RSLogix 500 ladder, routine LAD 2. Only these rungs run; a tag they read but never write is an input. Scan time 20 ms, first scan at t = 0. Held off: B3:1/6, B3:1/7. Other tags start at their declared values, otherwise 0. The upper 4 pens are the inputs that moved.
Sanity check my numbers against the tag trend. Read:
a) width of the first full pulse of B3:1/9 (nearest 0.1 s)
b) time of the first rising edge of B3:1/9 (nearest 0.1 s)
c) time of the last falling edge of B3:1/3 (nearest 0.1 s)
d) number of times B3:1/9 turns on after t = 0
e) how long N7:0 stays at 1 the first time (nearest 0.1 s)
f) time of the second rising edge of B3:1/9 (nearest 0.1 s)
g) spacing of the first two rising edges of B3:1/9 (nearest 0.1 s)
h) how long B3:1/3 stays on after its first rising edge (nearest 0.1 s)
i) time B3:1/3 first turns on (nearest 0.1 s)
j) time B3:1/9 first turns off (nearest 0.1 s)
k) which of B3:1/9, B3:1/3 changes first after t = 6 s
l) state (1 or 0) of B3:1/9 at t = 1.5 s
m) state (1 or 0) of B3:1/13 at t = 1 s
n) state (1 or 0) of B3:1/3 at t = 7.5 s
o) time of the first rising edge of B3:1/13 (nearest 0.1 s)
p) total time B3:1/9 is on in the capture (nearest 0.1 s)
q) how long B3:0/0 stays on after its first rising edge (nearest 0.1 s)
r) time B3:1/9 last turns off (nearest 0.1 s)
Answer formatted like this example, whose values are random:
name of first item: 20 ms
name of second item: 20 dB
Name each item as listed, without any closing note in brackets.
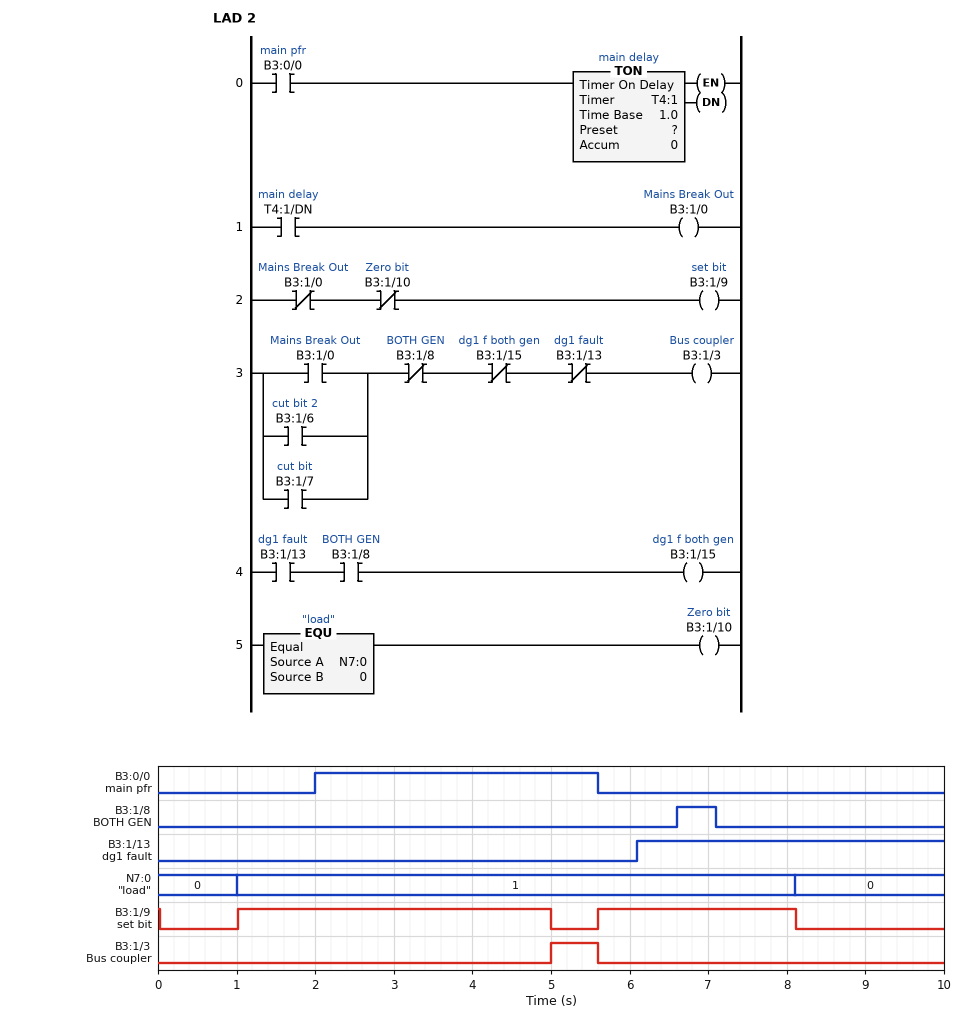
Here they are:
width of the first full pulse of B3:1/9: 4.0 s
time of the first rising edge of B3:1/9: 1.0 s
time of the last falling edge of B3:1/3: 5.6 s
number of times B3:1/9 turns on after t = 0: 2
how long N7:0 stays at 1 the first time: 7.1 s
time of the second rising edge of B3:1/9: 5.6 s
spacing of the first two rising edges of B3:1/9: 4.6 s
how long B3:1/3 stays on after its first rising edge: 0.6 s
time B3:1/3 first turns on: 5.0 s
time B3:1/9 first turns off: 0.0 s
which of B3:1/9, B3:1/3 changes first after t = 6 s: B3:1/9
state (1 or 0) of B3:1/9 at t = 1.5 s: 1
state (1 or 0) of B3:1/13 at t = 1 s: 0
state (1 or 0) of B3:1/3 at t = 7.5 s: 0
time of the first rising edge of B3:1/13: 6.1 s
total time B3:1/9 is on in the capture: 6.5 s
how long B3:0/0 stays on after its first rising edge: 3.6 s
time B3:1/9 last turns off: 8.1 s
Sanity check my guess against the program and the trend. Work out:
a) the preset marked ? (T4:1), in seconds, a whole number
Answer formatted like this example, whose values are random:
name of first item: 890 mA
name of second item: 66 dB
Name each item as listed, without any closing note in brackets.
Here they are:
the preset marked ? (T4:1), in seconds, a whole number: 3 s
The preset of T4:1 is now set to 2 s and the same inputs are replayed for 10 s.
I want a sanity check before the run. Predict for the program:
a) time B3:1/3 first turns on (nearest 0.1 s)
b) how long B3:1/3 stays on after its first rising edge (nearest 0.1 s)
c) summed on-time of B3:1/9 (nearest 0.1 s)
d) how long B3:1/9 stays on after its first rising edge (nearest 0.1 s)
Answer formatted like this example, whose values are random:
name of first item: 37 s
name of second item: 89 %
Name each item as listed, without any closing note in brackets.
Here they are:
time B3:1/3 first turns on: 4.0 s
how long B3:1/3 stays on after its first rising edge: 1.6 s
summed on-time of B3:1/9: 5.5 s
how long B3:1/9 stays on after its first rising edge: 3.0 s
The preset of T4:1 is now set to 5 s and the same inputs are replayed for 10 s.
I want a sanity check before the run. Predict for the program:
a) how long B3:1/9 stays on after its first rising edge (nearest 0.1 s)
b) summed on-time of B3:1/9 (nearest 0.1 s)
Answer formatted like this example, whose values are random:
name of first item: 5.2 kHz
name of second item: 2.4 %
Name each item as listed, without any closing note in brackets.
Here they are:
how long B3:1/9 stays on after its first rising edge: 7.1 s
summed on-time of B3:1/9: 7.1 s
